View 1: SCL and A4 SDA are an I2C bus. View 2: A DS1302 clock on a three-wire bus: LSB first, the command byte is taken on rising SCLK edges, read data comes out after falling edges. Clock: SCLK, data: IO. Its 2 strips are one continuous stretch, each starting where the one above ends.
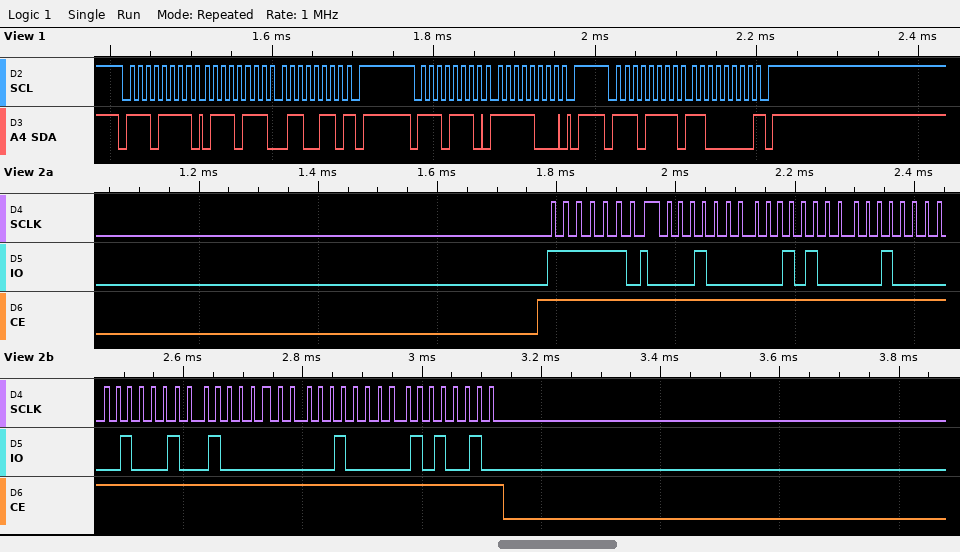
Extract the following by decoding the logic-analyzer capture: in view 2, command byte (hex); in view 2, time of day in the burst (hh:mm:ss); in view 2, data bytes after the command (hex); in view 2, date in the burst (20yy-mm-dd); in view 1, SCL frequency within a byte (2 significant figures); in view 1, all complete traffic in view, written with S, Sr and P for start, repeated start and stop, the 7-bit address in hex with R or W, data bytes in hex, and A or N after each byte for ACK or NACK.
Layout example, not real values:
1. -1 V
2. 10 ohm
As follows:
1. 0xBF
2. 04:14:08
3. 08 14 04 22 01 04 25
4. 2025-01-22
5. 100 kHz
6. S 77R A 77 A 66 N P S 77W A F8 A P S 77R A C0 N P
